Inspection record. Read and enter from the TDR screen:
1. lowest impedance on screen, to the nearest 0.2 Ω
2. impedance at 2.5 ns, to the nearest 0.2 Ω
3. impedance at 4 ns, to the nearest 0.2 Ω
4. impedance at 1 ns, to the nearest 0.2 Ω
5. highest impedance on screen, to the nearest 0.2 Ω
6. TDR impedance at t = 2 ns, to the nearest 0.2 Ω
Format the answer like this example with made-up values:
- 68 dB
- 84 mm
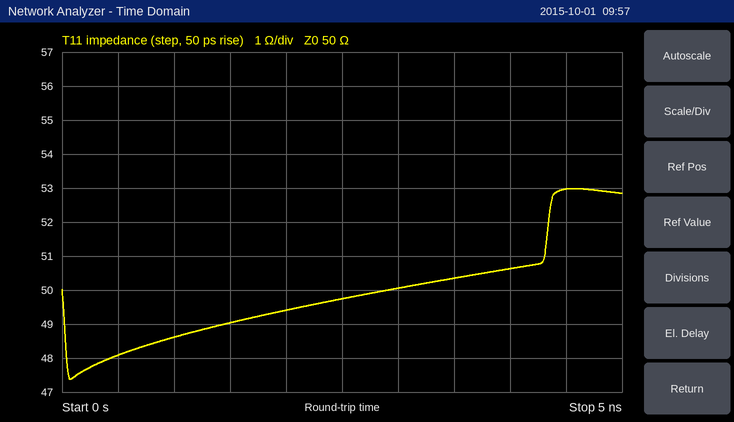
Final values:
- 47.4 Ω
- 49.8 Ω
- 50.6 Ω
- 48.6 Ω
- 53.0 Ω
- 49.4 Ω
